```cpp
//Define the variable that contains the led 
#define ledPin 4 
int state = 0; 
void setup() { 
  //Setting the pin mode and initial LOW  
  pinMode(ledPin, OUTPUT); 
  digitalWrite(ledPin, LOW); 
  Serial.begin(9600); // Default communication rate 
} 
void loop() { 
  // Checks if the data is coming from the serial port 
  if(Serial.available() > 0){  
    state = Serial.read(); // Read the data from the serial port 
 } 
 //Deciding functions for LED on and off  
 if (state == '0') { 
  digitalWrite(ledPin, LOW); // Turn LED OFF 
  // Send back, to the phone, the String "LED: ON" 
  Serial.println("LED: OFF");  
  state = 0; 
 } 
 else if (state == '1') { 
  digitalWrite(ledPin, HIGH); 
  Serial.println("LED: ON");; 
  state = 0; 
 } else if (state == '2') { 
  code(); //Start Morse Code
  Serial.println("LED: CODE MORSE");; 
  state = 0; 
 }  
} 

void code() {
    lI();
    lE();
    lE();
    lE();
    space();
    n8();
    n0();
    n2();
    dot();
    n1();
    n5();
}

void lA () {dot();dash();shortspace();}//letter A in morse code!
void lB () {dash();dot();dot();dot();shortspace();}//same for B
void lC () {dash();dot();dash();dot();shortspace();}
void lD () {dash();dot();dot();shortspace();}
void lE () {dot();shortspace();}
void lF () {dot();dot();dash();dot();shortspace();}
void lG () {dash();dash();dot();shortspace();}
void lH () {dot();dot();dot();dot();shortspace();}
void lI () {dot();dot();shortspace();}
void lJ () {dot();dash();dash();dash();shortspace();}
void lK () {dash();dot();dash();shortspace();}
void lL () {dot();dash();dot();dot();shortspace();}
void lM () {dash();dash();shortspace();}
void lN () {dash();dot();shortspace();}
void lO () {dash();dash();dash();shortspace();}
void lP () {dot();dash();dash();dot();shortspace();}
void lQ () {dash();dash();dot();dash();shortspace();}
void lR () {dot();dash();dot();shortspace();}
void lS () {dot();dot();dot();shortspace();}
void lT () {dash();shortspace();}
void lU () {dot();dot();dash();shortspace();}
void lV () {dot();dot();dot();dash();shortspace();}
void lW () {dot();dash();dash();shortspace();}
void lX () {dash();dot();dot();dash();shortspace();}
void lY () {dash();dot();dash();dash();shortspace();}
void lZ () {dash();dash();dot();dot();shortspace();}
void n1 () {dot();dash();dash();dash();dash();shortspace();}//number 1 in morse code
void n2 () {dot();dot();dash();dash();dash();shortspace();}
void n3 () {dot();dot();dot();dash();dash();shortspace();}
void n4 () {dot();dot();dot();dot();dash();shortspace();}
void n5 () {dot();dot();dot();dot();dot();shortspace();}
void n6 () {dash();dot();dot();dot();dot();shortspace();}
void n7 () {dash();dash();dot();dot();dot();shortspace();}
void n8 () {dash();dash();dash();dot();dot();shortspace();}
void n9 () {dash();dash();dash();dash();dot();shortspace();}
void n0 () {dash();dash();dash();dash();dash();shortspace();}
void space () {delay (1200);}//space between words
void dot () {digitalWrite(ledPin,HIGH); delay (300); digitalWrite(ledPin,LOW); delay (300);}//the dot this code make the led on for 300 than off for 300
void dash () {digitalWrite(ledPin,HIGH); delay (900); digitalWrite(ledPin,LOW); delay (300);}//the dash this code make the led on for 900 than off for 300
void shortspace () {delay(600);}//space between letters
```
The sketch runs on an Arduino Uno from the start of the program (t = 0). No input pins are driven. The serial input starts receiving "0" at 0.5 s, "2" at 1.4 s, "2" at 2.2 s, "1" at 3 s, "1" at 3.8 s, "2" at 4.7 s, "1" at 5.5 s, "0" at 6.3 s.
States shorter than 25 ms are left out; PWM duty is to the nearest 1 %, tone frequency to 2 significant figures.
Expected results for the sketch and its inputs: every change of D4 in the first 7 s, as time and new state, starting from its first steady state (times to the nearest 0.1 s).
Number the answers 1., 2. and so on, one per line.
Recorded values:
1. 0 s low; 1.4 s high; 1.7 s low; 2 s high; 2.3 s low; 3.2 s high; 3.5 s low; 4.4 s high; 4.7 s low; 5.6 s high; 5.9 s low
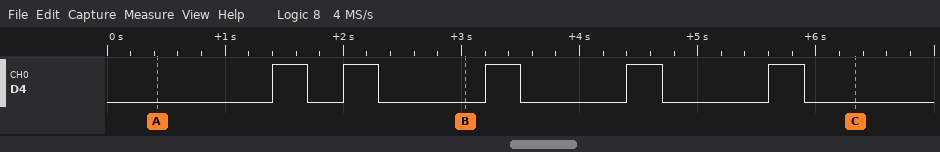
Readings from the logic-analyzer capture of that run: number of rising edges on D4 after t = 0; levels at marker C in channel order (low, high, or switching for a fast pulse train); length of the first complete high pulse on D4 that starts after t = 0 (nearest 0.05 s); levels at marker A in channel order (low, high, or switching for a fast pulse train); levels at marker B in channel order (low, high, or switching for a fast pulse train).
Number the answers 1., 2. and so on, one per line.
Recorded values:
1. 5
2. D4 low
3. 0.30 s
4. D4 low
5. D4 low
